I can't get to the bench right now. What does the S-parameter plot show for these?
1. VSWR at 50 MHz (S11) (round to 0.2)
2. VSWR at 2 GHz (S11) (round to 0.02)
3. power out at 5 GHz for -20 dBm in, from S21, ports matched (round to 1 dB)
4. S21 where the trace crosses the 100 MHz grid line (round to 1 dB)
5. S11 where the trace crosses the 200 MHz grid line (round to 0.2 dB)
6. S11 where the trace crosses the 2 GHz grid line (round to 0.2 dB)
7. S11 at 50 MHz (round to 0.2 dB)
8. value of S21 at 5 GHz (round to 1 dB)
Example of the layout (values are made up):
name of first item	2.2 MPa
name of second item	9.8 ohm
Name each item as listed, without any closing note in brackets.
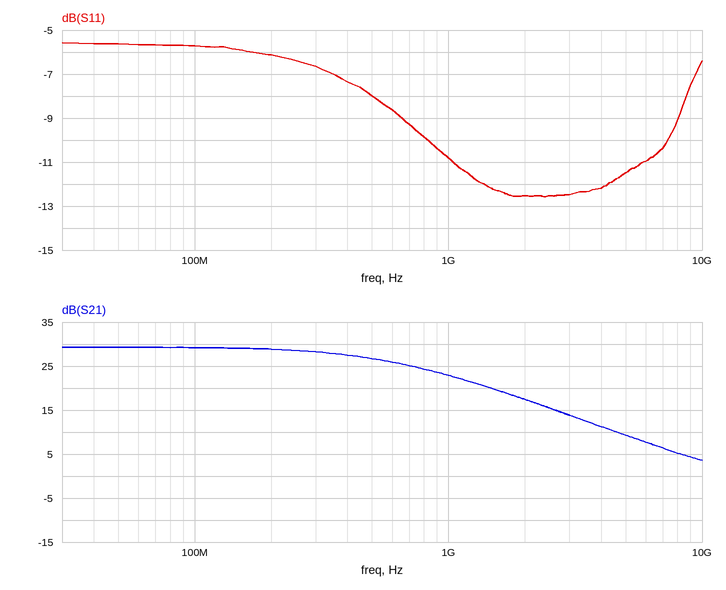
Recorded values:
VSWR at 50 MHz (S11)	3.2
VSWR at 2 GHz (S11)	1.62
power out at 5 GHz for -20 dBm in, from S21, ports matched	-11 dBm
S21 where the trace crosses the 100 MHz grid line	29 dB
S11 where the trace crosses the 200 MHz grid line	-6.2 dB
S11 where the trace crosses the 2 GHz grid line	-12.6 dB
S11 at 50 MHz	-5.6 dB
value of S21 at 5 GHz	9 dB
